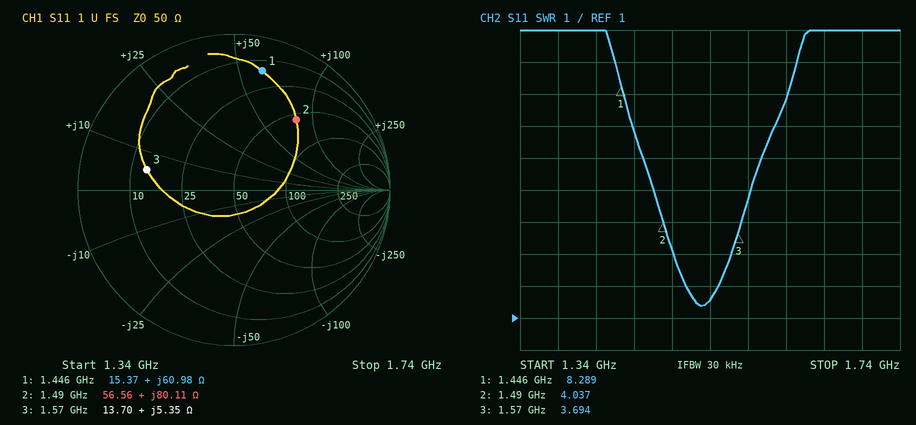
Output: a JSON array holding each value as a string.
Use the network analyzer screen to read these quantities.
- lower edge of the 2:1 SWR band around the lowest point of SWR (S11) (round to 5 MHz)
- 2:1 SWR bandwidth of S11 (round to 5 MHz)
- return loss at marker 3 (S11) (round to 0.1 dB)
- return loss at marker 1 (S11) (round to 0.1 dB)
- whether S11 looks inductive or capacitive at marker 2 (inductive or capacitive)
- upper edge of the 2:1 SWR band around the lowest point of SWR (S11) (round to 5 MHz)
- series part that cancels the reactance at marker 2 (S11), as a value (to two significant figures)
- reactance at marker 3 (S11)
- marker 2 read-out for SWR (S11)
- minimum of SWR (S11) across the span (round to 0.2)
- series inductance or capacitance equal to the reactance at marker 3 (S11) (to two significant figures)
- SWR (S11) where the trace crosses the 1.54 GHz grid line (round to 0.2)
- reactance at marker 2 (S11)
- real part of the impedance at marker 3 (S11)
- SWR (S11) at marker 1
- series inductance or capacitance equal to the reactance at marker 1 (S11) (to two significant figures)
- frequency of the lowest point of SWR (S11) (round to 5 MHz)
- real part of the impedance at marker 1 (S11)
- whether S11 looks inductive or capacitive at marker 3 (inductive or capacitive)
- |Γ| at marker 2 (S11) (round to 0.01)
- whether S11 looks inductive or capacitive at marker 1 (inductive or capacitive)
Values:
["1.515 GHz", "35 MHz", "4.8 dB", "2.1 dB", "inductive", "1.550 GHz", "1.3 pF", "+5.35 Ω", "4.037", "1.4", "540 pH", "1.6", "+80.11 Ω", "13.70 Ω", "8.289", "6.7 nH", "1.530 GHz", "15.37 Ω", "inductive", "0.60", "inductive"]
